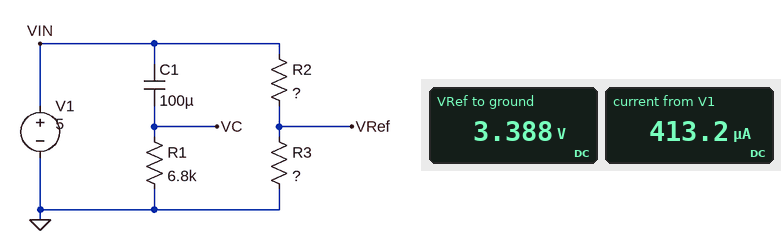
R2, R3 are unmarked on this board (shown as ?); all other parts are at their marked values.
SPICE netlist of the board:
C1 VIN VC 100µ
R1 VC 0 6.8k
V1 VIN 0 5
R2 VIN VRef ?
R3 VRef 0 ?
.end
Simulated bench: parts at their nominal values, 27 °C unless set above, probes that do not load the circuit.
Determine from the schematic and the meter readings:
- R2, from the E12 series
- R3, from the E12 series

3.9 kΩ
8.2 kΩ
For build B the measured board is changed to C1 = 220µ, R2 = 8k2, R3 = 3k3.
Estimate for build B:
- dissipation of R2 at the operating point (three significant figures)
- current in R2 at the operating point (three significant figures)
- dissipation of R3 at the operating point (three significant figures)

1.55 mW
435 µA
624 µW
